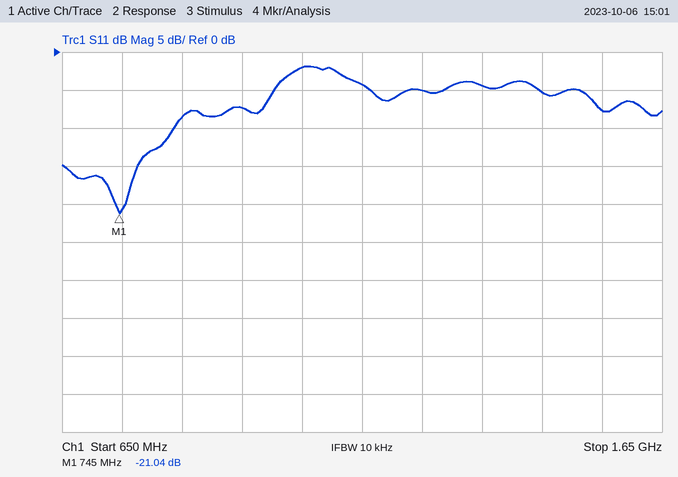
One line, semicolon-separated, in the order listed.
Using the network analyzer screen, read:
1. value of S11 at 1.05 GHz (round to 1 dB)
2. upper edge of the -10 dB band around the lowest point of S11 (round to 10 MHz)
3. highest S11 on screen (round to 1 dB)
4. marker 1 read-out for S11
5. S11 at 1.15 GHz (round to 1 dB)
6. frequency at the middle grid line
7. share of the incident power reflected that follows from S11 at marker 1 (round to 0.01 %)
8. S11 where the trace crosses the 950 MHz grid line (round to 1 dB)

-2 dB; 840 MHz; -2 dB; -21.04 dB; -4 dB; 1.15 GHz; 0.79 %; -7 dB
